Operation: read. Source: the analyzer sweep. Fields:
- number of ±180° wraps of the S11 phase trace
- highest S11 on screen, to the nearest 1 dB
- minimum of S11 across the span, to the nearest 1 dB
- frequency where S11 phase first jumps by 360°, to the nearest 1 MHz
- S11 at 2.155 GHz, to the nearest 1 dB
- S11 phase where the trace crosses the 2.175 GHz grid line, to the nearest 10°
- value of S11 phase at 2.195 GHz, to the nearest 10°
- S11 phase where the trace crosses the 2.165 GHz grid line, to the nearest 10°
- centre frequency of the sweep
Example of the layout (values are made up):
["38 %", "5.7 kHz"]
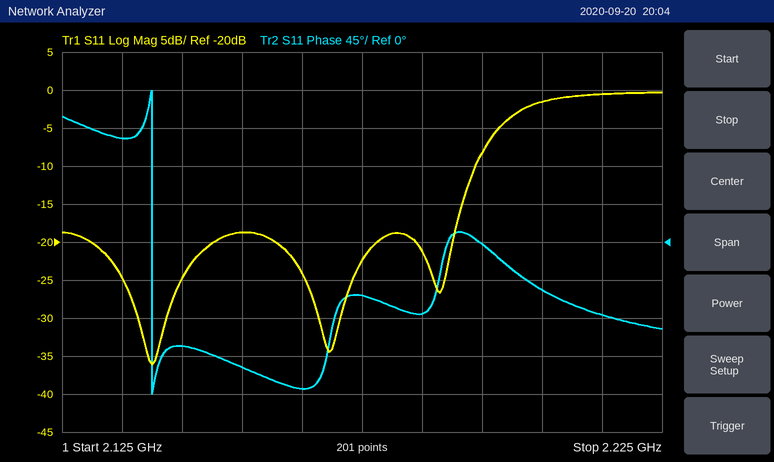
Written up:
["1", "0 dB", "-36 dB", "2.140 GHz", "-19 dB", "-60°", "0°", "-170°", "2.175 GHz"]
